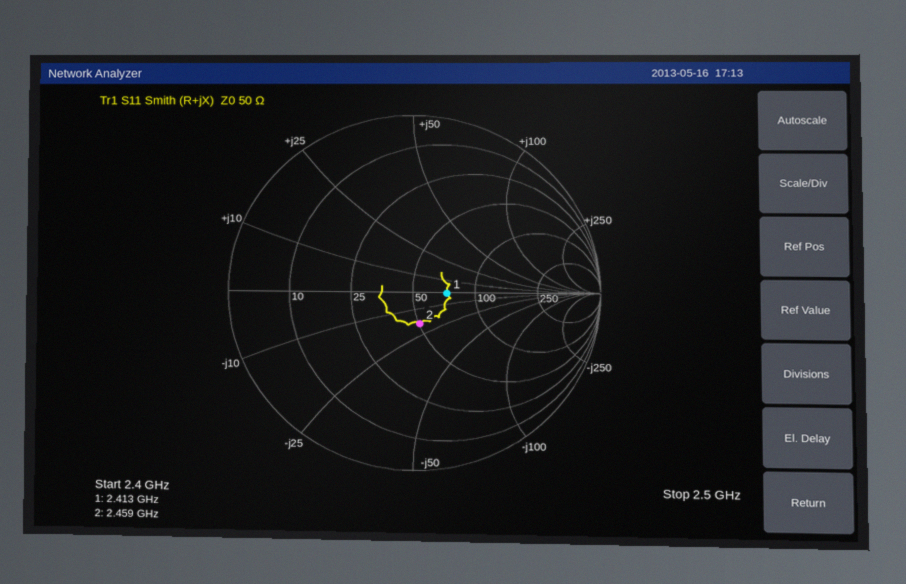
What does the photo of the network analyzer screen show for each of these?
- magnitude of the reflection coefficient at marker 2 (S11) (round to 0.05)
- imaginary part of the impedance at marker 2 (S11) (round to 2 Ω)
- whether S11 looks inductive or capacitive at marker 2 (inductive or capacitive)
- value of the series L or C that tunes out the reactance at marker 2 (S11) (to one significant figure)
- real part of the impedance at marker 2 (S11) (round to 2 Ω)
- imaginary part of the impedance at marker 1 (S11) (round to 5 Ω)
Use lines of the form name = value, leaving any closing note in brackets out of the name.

magnitude of the reflection coefficient at marker 2 (S11) = 0.20
imaginary part of the impedance at marker 2 (S11) = -18 Ω
whether S11 looks inductive or capacitive at marker 2 = capacitive
value of the series L or C that tunes out the reactance at marker 2 (S11) = 1 nH
real part of the impedance at marker 2 (S11) = 50 Ω
imaginary part of the impedance at marker 1 (S11) = 0 Ω
